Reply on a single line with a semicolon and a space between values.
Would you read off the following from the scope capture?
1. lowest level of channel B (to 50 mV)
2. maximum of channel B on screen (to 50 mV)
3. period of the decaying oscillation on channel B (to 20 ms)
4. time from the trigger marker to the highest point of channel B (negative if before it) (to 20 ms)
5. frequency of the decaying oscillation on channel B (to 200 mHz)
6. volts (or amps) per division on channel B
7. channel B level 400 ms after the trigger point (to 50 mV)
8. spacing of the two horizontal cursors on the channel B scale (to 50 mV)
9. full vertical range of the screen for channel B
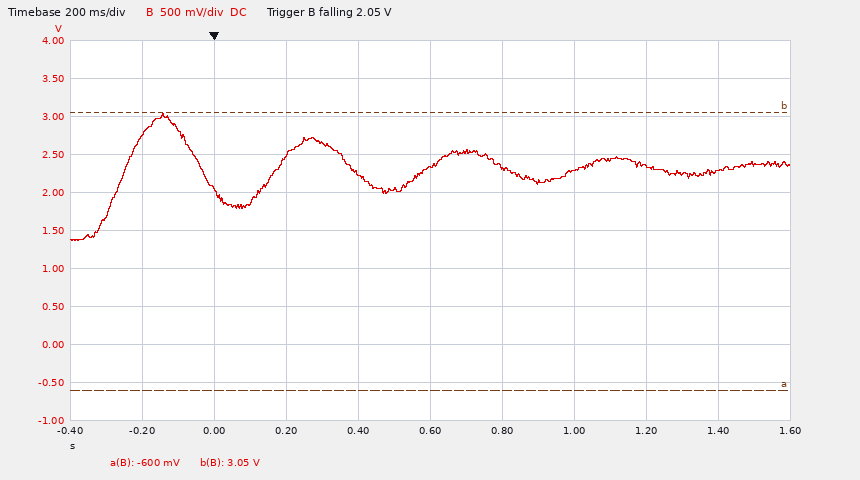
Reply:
1.35 V; 3.05 V; 420 ms; -140 ms; 2.4 Hz; 500 mV; 2.25 V; 3.65 V; 5 V
